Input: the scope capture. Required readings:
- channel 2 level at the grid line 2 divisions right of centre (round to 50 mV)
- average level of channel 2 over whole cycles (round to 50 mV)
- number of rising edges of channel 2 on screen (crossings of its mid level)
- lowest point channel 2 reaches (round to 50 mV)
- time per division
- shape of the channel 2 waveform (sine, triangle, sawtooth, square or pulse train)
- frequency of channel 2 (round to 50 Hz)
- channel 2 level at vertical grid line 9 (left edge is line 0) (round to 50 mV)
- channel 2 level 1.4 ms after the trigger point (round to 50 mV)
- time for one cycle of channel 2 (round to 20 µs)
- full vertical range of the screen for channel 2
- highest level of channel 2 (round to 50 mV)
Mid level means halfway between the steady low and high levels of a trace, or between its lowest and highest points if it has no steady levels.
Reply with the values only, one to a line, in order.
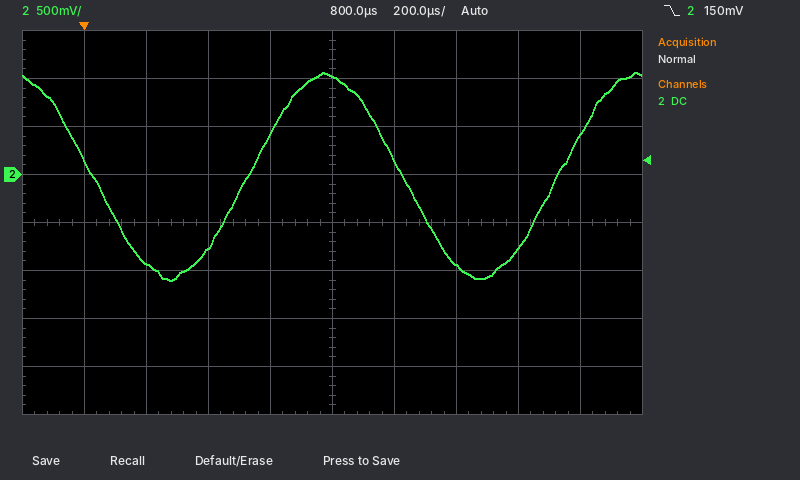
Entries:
-950 mV
0 mV
2
-1.10 V
200 µs
sine
1.00 kHz
400 mV
-750 mV
1.00 ms
4 V
1.05 V
